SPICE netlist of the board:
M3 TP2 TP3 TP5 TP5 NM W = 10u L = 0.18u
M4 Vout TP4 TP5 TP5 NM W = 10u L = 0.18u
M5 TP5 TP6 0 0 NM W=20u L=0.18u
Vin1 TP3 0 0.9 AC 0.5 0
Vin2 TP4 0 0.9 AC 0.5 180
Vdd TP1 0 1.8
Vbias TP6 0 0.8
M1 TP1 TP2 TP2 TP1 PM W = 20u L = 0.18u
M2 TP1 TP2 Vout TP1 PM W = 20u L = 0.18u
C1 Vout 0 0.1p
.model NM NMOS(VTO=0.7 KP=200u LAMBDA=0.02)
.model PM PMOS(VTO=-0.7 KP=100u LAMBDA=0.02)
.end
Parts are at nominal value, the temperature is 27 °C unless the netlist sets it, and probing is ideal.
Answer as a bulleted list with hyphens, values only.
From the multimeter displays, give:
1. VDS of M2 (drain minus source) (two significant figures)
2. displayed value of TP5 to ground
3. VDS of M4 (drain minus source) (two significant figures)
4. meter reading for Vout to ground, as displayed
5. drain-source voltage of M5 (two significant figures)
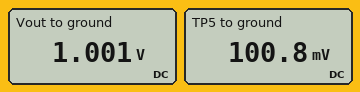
- 800 mV
- 100.8 mV
- 900 mV
- 1.001 V
- 100 mV
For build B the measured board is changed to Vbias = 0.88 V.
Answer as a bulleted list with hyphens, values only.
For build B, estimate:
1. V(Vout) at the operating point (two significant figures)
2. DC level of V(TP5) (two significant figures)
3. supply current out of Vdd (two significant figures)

- 960 mV
- 64 mV
- 210 µA
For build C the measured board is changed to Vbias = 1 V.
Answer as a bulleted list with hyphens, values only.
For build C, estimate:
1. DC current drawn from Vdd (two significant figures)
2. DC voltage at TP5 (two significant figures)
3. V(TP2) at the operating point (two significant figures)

- 270 µA
- 44 mV
- 940 mV
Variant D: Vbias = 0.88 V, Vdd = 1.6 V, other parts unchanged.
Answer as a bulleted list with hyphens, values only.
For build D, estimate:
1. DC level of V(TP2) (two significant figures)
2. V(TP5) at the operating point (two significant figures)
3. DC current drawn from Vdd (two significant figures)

- 760 mV
- 64 mV
- 210 µA
